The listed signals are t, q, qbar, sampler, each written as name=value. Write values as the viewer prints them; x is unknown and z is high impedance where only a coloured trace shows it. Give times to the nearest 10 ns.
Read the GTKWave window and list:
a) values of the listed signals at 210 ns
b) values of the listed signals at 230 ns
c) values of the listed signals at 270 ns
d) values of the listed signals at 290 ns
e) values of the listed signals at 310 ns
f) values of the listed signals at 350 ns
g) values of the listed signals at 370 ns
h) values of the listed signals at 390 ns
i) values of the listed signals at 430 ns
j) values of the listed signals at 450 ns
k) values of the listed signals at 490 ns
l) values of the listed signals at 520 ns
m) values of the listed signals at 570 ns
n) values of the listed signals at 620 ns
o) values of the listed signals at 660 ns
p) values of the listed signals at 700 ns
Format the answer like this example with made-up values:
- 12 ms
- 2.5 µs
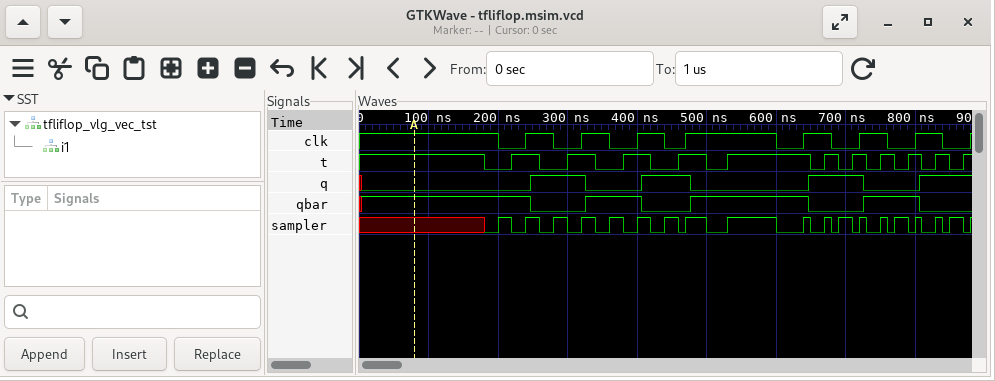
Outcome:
- t=0, q=0, qbar=1, sampler=1
- t=1, q=0, qbar=1, sampler=0
- t=0, q=1, qbar=0, sampler=0
- t=0, q=1, qbar=0, sampler=1
- t=1, q=1, qbar=0, sampler=0
- t=0, q=0, qbar=1, sampler=0
- t=0, q=0, qbar=1, sampler=1
- t=1, q=0, qbar=1, sampler=0
- t=0, q=1, qbar=0, sampler=0
- t=0, q=1, qbar=0, sampler=1
- t=1, q=0, qbar=1, sampler=1
- t=0, q=0, qbar=1, sampler=0
- t=1, q=0, qbar=1, sampler=1
- t=1, q=0, qbar=1, sampler=0
- t=0, q=1, qbar=0, sampler=0
- t=0, q=1, qbar=0, sampler=1
